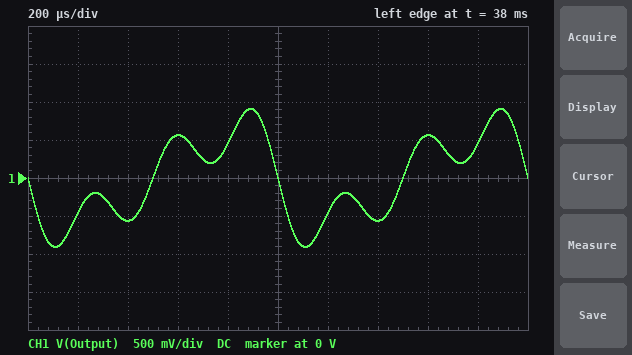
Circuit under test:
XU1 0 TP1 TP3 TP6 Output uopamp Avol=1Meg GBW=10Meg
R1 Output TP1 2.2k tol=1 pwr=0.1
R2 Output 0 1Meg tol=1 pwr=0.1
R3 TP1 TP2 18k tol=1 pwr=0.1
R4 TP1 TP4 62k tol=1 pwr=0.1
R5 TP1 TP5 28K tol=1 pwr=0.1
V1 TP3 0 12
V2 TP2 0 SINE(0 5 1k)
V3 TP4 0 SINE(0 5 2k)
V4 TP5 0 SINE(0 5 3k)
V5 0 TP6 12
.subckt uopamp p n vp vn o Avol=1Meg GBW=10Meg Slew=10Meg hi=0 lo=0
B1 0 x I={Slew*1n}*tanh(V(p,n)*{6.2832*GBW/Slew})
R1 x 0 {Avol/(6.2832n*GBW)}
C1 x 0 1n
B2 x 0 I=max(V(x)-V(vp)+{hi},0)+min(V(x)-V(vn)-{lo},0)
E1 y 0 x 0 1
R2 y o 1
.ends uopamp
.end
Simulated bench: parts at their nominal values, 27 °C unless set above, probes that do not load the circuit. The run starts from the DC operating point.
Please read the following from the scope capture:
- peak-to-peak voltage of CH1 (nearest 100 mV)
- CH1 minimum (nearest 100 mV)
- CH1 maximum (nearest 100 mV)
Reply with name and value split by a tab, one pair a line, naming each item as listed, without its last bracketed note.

peak-to-peak voltage of CH1	1.8 V
CH1 minimum	-900 mV
CH1 maximum	900 mV
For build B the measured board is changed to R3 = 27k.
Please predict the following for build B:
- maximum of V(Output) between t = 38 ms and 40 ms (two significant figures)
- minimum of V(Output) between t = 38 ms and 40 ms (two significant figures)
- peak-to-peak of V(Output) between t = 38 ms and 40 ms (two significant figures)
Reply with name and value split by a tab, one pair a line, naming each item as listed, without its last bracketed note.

maximum of V(Output) between t = 38 ms and 40 ms	780 mV
minimum of V(Output) between t = 38 ms and 40 ms	-780 mV
peak-to-peak of V(Output) between t = 38 ms and 40 ms	1.6 V
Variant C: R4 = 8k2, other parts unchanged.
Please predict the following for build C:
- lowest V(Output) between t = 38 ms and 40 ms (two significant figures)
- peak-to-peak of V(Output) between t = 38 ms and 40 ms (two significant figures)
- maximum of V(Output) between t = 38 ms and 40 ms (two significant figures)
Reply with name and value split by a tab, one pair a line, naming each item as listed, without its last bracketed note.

lowest V(Output) between t = 38 ms and 40 ms	-2.1 V
peak-to-peak of V(Output) between t = 38 ms and 40 ms	4.1 V
maximum of V(Output) between t = 38 ms and 40 ms	2.1 V
